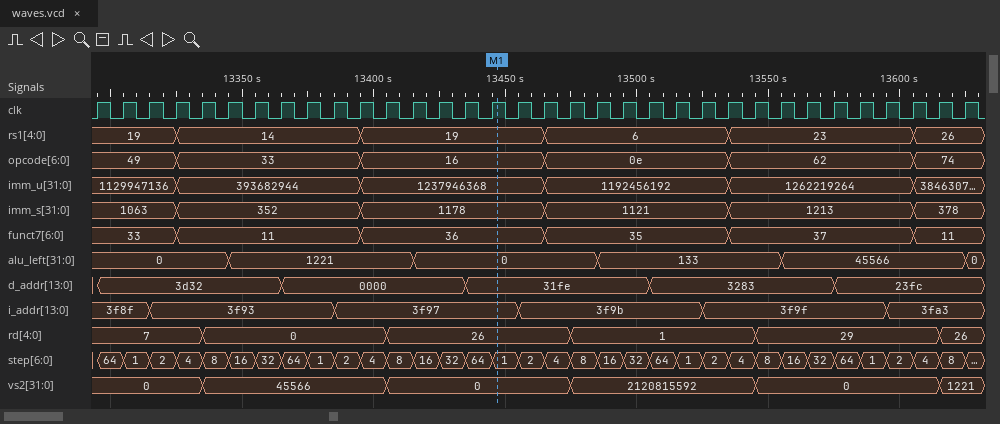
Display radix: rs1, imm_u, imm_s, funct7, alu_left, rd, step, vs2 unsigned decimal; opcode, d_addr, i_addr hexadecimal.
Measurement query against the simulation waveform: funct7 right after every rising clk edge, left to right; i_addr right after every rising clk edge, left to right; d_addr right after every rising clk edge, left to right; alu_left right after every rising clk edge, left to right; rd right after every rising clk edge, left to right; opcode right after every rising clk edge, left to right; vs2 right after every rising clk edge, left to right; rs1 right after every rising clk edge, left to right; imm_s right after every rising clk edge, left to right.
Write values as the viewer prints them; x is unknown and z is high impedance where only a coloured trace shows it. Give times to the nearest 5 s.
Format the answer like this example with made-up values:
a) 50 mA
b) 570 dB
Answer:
a) 33, 33, 33, 11, 11, 11, 11, 11, 11, 11, 36, 36, 36, 36, 36, 36, 36, 35, 35, 35, 35, 35, 35, 35, 37, 37, 37, 37, 37, 37, 37, 11, 11, 11
b) 3f8f, 3f8f, 3f93, 3f93, 3f93, 3f93, 3f93, 3f93, 3f93, 3f97, 3f97, 3f97, 3f97, 3f97, 3f97, 3f97, 3f9b, 3f9b, 3f9b, 3f9b, 3f9b, 3f9b, 3f9b, 3f9f, 3f9f, 3f9f, 3f9f, 3f9f, 3f9f, 3f9f, 3fa3, 3fa3, 3fa3, 3fa3
c) 3d32, 3d32, 3d32, 3d32, 3d32, 3d32, 3d32, 0000, 0000, 0000, 0000, 0000, 0000, 0000, 31fe, 31fe, 31fe, 31fe, 31fe, 31fe, 31fe, 3283, 3283, 3283, 3283, 3283, 3283, 3283, 23fc, 23fc, 23fc, 23fc, 23fc, 23fc
d) 0, 0, 0, 0, 0, 1221, 1221, 1221, 1221, 1221, 1221, 1221, 0, 0, 0, 0, 0, 0, 0, 133, 133, 133, 133, 133, 133, 133, 45566, 45566, 45566, 45566, 45566, 45566, 45566, 0
e) 7, 7, 7, 7, 0, 0, 0, 0, 0, 0, 0, 26, 26, 26, 26, 26, 26, 26, 1, 1, 1, 1, 1, 1, 1, 29, 29, 29, 29, 29, 29, 29, 26, 26
f) 49, 49, 49, 33, 33, 33, 33, 33, 33, 33, 16, 16, 16, 16, 16, 16, 16, 0e, 0e, 0e, 0e, 0e, 0e, 0e, 62, 62, 62, 62, 62, 62, 62, 74, 74, 74
g) 0, 0, 0, 0, 45566, 45566, 45566, 45566, 45566, 45566, 45566, 0, 0, 0, 0, 0, 0, 0, 2120815592, 2120815592, 2120815592, 2120815592, 2120815592, 2120815592, 2120815592, 0, 0, 0, 0, 0, 0, 0, 1221, 1221
h) 19, 19, 19, 14, 14, 14, 14, 14, 14, 14, 19, 19, 19, 19, 19, 19, 19, 6, 6, 6, 6, 6, 6, 6, 23, 23, 23, 23, 23, 23, 23, 26, 26, 26
i) 1063, 1063, 1063, 352, 352, 352, 352, 352, 352, 352, 1178, 1178, 1178, 1178, 1178, 1178, 1178, 1121, 1121, 1121, 1121, 1121, 1121, 1121, 1213, 1213, 1213, 1213, 1213, 1213, 1213, 378, 378, 378
